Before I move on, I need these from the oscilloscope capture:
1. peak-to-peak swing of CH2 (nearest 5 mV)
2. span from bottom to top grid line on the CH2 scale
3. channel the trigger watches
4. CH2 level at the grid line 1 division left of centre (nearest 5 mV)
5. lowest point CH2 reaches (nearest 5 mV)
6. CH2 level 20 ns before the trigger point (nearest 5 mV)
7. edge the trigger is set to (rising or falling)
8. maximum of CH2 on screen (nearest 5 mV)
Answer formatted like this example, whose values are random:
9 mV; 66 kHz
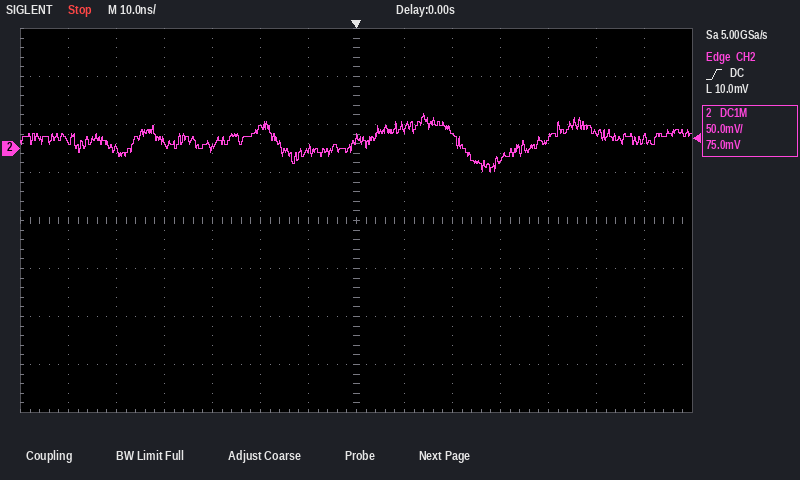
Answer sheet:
60 mV; 400 mV; CH2; 0 mV; -25 mV; 20 mV; rising; 35 mV
